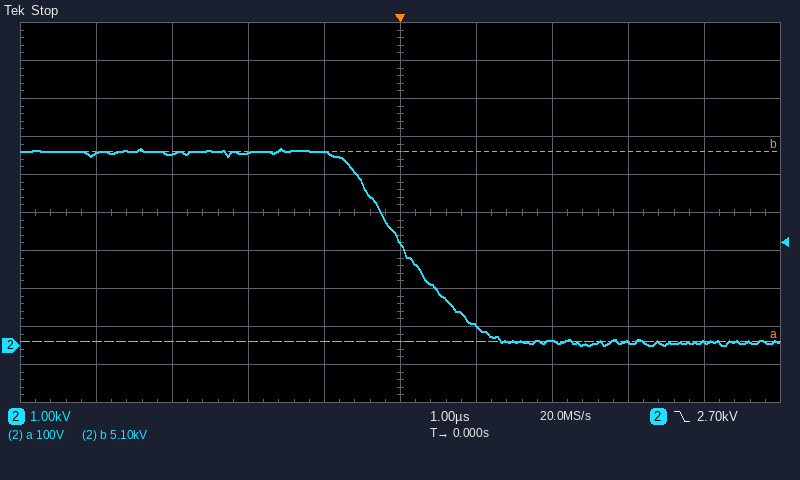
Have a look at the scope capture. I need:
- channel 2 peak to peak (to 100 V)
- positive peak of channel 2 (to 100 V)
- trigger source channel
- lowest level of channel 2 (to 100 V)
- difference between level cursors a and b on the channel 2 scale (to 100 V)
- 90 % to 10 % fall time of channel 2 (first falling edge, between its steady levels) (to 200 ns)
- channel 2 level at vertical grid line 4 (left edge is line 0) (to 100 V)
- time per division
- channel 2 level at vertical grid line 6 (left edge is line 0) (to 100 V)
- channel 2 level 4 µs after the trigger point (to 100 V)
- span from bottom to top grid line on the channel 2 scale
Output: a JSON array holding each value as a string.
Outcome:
["5.2 kV", "5.2 kV", "channel 2", "0.0 kV", "5.0 kV", "1.6 µs", "5.1 kV", "1 µs", "500 V", "100 V", "10 kV"]
